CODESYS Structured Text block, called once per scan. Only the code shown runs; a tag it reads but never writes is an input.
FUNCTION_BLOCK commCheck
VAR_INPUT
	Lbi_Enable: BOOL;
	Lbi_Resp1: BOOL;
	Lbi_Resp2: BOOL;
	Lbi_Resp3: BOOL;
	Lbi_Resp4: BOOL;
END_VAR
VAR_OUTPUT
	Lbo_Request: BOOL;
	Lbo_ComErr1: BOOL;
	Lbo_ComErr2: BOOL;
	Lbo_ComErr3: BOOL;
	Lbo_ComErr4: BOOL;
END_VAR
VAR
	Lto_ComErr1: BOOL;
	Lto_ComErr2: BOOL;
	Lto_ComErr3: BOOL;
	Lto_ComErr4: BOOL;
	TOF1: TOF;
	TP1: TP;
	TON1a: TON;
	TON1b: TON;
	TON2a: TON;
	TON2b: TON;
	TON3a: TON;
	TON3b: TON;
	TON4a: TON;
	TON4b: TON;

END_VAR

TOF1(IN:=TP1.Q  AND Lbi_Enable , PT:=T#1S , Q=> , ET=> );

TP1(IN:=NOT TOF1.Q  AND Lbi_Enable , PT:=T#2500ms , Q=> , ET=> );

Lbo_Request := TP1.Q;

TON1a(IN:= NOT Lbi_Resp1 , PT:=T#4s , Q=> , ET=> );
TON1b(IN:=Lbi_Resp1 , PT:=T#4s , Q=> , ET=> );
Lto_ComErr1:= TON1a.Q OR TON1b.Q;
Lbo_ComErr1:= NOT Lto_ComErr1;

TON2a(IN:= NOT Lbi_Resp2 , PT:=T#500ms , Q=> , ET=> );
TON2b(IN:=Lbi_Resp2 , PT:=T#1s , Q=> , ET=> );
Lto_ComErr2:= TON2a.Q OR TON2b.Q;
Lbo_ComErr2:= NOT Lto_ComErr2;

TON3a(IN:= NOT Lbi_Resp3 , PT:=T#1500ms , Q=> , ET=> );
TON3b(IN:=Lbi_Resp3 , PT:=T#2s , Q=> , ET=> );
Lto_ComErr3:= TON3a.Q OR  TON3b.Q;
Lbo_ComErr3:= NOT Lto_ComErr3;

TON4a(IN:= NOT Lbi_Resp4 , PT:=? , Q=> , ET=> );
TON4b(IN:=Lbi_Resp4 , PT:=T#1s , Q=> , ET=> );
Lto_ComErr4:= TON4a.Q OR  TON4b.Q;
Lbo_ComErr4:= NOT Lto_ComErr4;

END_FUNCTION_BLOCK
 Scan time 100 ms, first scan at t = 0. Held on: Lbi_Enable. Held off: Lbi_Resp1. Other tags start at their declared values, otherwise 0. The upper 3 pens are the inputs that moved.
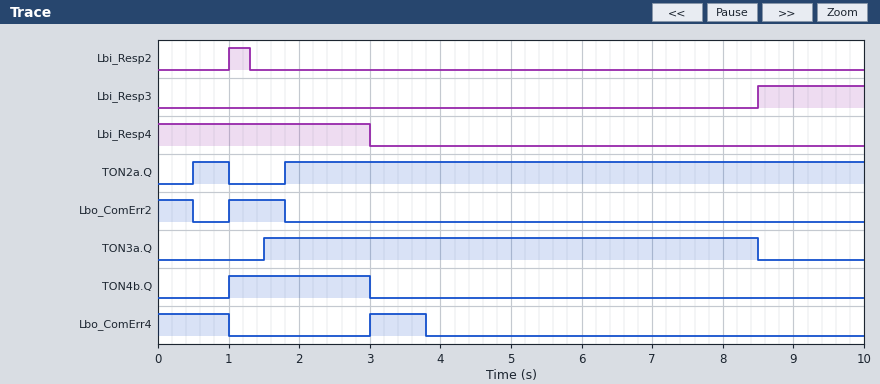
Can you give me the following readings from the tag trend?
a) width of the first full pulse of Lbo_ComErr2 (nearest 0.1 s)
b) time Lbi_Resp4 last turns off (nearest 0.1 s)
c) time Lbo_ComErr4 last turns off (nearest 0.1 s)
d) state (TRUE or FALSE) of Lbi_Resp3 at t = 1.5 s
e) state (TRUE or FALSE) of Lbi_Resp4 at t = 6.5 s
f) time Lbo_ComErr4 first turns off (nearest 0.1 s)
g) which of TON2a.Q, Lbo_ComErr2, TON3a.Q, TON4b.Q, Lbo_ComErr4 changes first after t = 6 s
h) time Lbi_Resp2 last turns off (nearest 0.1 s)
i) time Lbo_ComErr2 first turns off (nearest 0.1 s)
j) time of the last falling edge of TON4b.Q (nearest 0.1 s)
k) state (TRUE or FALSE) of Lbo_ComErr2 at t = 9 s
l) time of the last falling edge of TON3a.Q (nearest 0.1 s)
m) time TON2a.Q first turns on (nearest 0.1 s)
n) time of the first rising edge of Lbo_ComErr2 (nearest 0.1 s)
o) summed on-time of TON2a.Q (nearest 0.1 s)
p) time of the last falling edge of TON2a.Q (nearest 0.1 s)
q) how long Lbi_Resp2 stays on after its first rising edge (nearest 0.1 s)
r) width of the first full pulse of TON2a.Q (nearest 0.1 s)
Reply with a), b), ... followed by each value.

a) 0.8 s
b) 3.0 s
c) 3.8 s
d) FALSE
e) FALSE
f) 1.0 s
g) TON3a.Q
h) 1.3 s
i) 0.5 s
j) 3.0 s
k) FALSE
l) 8.5 s
m) 0.5 s
n) 1.0 s
o) 8.7 s
p) 1.0 s
q) 0.3 s
r) 0.5 s
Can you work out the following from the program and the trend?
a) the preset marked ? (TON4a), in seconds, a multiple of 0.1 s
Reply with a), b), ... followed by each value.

a) 0.8 s
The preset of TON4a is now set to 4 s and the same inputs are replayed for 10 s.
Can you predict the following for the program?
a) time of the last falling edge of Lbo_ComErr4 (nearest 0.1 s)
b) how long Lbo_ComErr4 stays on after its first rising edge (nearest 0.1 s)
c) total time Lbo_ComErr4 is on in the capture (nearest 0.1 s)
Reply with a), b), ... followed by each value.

a) 7.0 s
b) 4.0 s
c) 5.0 s
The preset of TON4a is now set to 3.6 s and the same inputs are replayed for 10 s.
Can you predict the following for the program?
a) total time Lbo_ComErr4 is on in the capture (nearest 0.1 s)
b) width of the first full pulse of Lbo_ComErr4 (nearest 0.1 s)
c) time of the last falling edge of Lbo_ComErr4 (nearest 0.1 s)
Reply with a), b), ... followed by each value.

a) 4.6 s
b) 3.6 s
c) 6.6 s
